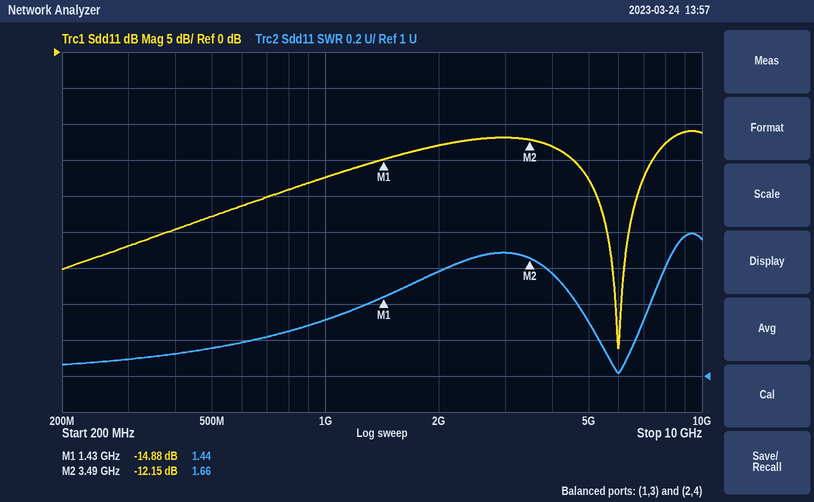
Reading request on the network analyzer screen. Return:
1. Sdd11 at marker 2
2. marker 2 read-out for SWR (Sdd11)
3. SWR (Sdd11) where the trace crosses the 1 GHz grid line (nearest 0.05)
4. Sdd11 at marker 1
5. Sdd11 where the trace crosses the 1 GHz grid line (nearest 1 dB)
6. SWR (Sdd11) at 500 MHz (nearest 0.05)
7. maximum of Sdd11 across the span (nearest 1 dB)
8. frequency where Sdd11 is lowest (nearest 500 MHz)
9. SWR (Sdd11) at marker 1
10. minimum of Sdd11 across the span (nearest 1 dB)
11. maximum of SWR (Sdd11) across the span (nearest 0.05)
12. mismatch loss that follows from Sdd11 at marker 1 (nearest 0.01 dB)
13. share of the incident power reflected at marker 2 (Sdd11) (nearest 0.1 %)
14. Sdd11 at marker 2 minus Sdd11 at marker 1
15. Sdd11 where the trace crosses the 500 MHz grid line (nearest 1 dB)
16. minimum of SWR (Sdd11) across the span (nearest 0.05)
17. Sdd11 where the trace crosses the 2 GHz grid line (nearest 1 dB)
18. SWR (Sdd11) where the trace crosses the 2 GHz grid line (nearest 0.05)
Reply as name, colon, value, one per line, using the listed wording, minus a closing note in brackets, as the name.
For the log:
Sdd11 at marker 2: -12.15 dB
marker 2 read-out for SWR: 1.66
SWR (Sdd11) where the trace crosses the 1 GHz grid line: 1.30
Sdd11 at marker 1: -14.88 dB
Sdd11 where the trace crosses the 1 GHz grid line: -17 dB
SWR (Sdd11) at 500 MHz: 1.15
maximum of Sdd11 across the span: -11 dB
frequency where Sdd11 is lowest: 6.0 GHz
SWR (Sdd11) at marker 1: 1.44
minimum of Sdd11 across the span: -41 dB
maximum of SWR (Sdd11) across the span: 1.80
mismatch loss that follows from Sdd11 at marker 1: 0.14 dB
share of the incident power reflected at marker 2 (Sdd11): 6.1 %
Sdd11 at marker 2 minus Sdd11 at marker 1: 2.73 dB
Sdd11 where the trace crosses the 500 MHz grid line: -23 dB
minimum of SWR (Sdd11) across the span: 1.00
Sdd11 where the trace crosses the 2 GHz grid line: -13 dB
SWR (Sdd11) where the trace crosses the 2 GHz grid line: 1.60
